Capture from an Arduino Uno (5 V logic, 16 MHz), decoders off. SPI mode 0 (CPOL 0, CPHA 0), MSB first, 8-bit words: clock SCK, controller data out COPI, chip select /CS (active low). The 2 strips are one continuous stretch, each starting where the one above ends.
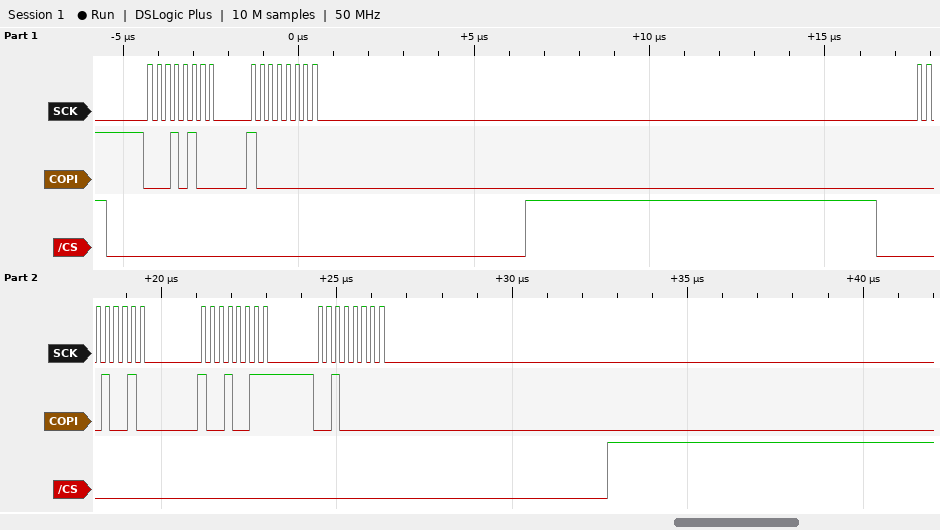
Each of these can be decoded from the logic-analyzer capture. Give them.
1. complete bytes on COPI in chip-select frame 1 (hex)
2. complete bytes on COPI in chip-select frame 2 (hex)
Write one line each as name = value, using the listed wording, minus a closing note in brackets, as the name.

complete bytes on COPI in chip-select frame 1 = 14 80
complete bytes on COPI in chip-select frame 2 = 12 93 20
